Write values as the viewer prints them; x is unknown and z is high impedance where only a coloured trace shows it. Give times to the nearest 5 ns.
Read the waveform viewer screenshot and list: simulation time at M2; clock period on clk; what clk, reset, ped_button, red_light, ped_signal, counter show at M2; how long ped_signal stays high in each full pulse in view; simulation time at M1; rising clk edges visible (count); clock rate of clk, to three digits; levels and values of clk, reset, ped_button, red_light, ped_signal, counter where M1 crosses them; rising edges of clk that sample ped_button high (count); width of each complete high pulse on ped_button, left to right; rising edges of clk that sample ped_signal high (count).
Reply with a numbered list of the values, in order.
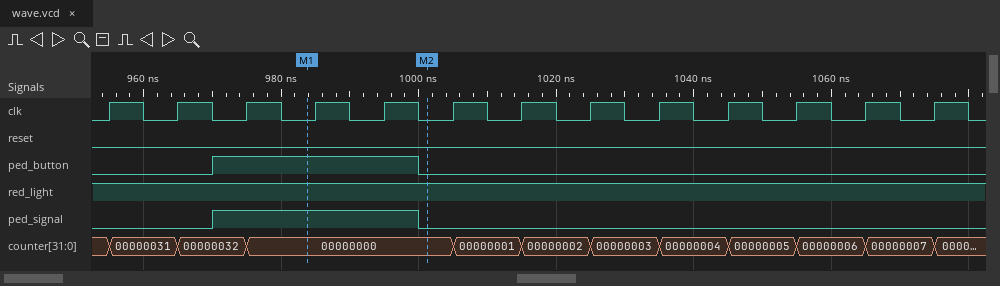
1. 1000 ns
2. 10 ns
3. clk=0, reset=0, ped_button=0, red_light=1, ped_signal=0, counter=00000000
4. 30 ns
5. 985 ns
6. 13
7. 100 MHz
8. clk=0, reset=0, ped_button=1, red_light=1, ped_signal=1, counter=00000000
9. 3
10. 30 ns
11. 3
